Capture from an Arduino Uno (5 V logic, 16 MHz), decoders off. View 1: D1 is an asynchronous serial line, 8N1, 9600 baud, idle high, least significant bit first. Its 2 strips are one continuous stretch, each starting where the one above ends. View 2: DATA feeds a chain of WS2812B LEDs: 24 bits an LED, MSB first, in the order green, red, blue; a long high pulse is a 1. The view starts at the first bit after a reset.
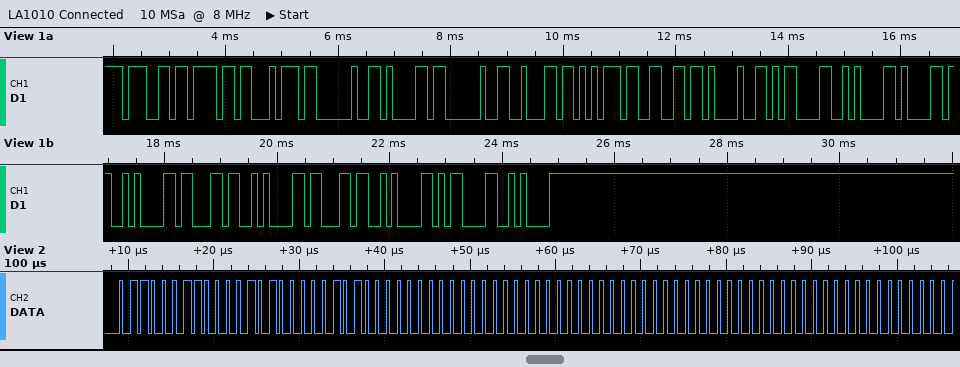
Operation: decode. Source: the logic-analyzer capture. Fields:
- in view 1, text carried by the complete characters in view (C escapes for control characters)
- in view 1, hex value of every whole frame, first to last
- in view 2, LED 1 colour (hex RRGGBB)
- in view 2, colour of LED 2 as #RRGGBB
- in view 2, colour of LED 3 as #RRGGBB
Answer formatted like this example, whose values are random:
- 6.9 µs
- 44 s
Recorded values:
- "got a buf!\r\na\nc\nc\n\r\n"
- 67 6F 74 20 61 20 62 75 66 21 0D 0A 61 0A 63 0A 63 0A 0D 0A
- #0A630A
- #000000
- #000000
